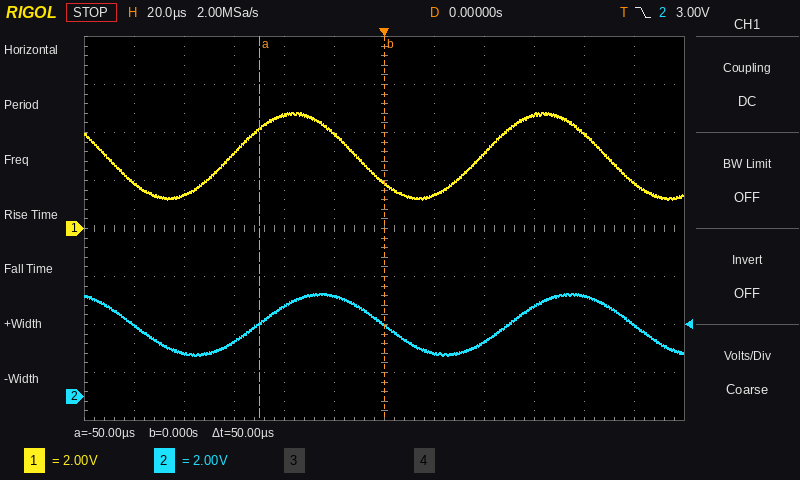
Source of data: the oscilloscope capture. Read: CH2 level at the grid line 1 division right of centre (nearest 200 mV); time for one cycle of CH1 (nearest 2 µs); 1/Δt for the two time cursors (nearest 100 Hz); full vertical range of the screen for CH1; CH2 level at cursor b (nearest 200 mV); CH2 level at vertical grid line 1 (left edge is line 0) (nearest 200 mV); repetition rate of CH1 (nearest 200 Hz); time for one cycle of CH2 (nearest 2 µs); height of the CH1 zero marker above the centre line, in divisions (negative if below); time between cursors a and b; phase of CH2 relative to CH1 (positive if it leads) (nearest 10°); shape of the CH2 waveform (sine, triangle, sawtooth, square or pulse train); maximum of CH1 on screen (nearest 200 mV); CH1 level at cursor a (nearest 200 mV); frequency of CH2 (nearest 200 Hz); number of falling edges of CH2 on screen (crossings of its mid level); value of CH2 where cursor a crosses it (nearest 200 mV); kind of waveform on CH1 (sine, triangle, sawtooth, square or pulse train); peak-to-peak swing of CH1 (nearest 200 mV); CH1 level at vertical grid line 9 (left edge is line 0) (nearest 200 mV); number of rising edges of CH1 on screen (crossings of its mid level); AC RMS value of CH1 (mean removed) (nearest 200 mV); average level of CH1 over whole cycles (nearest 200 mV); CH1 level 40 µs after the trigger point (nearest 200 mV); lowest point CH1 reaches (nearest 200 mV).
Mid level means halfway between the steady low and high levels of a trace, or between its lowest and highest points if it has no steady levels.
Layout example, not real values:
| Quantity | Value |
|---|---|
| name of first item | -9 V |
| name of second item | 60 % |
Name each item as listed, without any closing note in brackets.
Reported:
| Quantity | Value |
|---|---|
| CH2 level at the grid line 1 division right of centre | 1.8 V |
| time for one cycle of CH1 | 100 µs |
| 1/Δt for the two time cursors | 20.0 kHz |
| full vertical range of the screen for CH1 | 16 V |
| CH2 level at cursor b | 3.0 V |
| CH2 level at vertical grid line 1 (left edge is line 0) | 3.0 V |
| repetition rate of CH1 | 10.0 kHz |
| time for one cycle of CH2 | 100 µs |
| height of the CH1 zero marker above the centre line, in divisions | 0.0 div |
| time between cursors a and b | 50 µs |
| phase of CH2 relative to CH1 (positive if it leads) | -40° |
| shape of the CH2 waveform | sine |
| maximum of CH1 on screen | 4.8 V |
| CH1 level at cursor a | 4.2 V |
| frequency of CH2 | 10.0 kHz |
| number of falling edges of CH2 on screen | 3 |
| value of CH2 where cursor a crosses it | 3.0 V |
| kind of waveform on CH1 | sine |
| peak-to-peak swing of CH1 | 3.6 V |
| CH1 level at vertical grid line 9 (left edge is line 0) | 4.8 V |
| number of rising edges of CH1 on screen | 2 |
| AC RMS value of CH1 (mean removed) | 1.2 V |
| average level of CH1 over whole cycles | 3.0 V |
| CH1 level 40 µs after the trigger point | 3.2 V |
| lowest point CH1 reaches | 1.2 V |
